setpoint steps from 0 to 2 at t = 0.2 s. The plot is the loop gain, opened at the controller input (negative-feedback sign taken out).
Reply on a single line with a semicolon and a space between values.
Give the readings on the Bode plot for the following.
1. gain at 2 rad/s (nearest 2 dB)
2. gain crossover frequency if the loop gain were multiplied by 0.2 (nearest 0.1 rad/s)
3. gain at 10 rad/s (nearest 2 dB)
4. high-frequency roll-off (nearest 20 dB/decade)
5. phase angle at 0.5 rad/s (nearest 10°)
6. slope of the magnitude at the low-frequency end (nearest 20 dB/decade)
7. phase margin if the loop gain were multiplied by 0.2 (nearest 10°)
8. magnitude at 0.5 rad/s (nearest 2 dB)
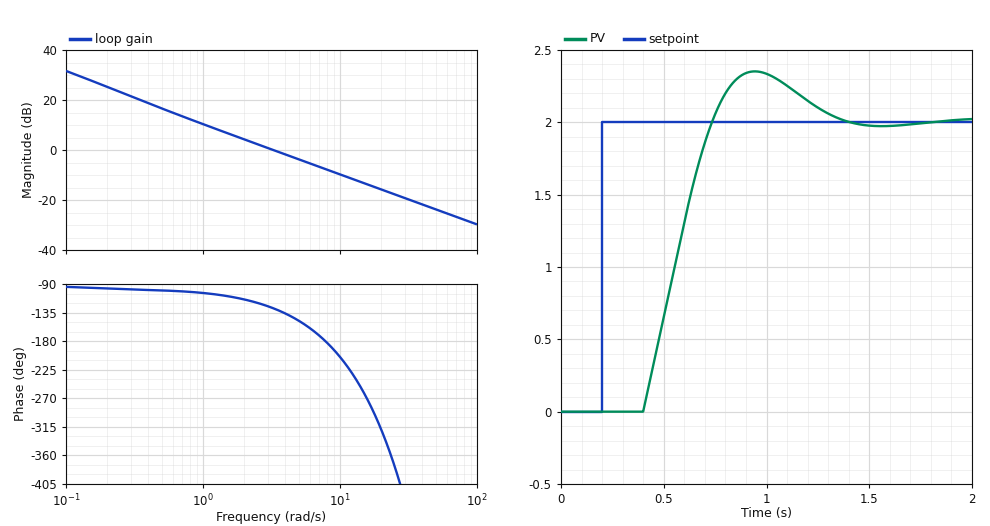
4 dB; 0.7 rad/s; -10 dB; -20 dB/decade; -100°; -20 dB/decade; 80°; 16 dB
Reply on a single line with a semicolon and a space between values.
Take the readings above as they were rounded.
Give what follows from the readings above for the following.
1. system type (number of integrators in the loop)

1
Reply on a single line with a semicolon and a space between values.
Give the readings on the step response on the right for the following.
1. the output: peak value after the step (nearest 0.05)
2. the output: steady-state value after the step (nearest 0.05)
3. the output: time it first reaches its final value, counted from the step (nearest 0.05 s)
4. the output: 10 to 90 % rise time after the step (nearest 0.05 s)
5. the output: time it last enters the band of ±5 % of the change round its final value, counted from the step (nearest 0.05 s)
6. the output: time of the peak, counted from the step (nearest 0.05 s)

2.35; 2.00; 0.55 s; 0.25 s; 1.05 s; 0.75 s
